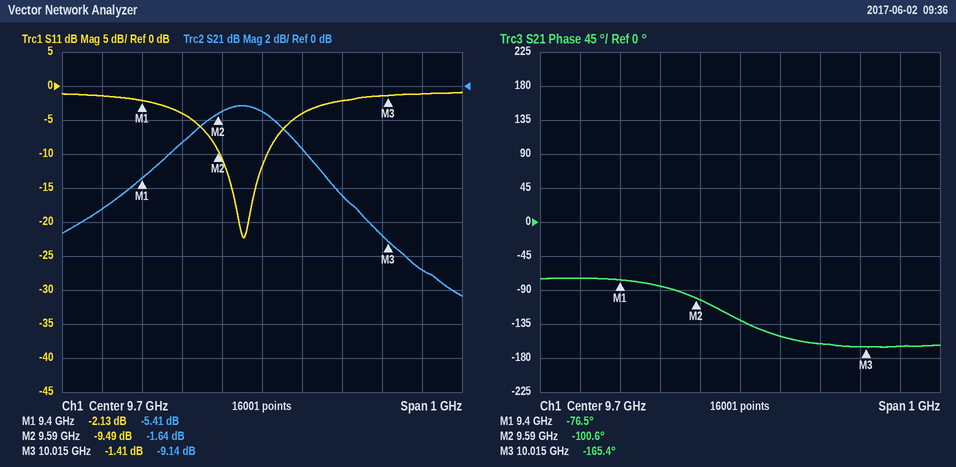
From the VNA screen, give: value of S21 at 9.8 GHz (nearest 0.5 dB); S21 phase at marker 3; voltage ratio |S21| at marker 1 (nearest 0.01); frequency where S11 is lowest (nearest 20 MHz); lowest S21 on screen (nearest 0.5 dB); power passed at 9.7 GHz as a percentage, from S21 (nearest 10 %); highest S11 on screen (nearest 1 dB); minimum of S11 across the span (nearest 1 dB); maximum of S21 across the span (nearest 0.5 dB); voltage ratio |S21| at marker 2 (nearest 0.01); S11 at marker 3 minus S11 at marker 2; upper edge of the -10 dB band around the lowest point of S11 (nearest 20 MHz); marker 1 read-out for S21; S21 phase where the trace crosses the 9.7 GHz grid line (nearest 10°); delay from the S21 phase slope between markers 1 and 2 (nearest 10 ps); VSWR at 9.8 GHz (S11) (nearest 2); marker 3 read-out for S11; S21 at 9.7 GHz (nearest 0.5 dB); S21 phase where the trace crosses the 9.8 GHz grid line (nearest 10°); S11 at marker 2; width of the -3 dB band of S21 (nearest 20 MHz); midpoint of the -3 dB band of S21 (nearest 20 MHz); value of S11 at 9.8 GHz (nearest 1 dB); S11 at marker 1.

-3.5 dB
-165.4°
0.54
9.66 GHz
-12.5 dB
70 %
-1 dB
-22 dB
-1.0 dB
0.83
8.08 dB
9.72 GHz
-5.41 dB
-130°
350 ps
4
-1.41 dB
-1.5 dB
-150°
-9.49 dB
360 MHz
9.64 GHz
-4 dB
-2.13 dB
